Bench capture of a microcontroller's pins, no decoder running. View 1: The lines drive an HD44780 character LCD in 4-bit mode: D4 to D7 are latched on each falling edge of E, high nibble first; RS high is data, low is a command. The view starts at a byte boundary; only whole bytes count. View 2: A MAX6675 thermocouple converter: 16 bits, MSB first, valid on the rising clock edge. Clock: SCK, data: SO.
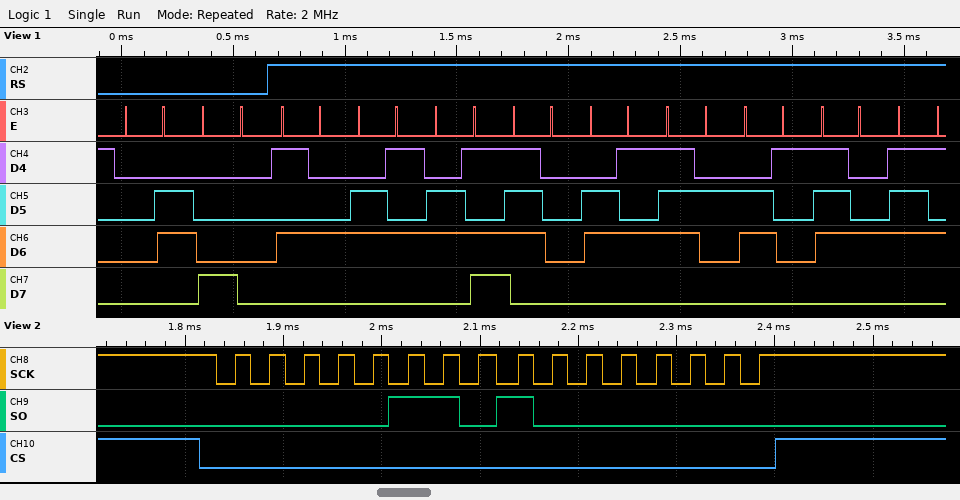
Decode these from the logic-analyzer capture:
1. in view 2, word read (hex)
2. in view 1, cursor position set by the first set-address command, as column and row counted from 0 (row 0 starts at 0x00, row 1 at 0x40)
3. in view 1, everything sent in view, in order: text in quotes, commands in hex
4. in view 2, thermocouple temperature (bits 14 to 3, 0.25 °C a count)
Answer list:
0x0680
column 0, row 0
0x06 0x80 "Temperatu"
52.00 °C
